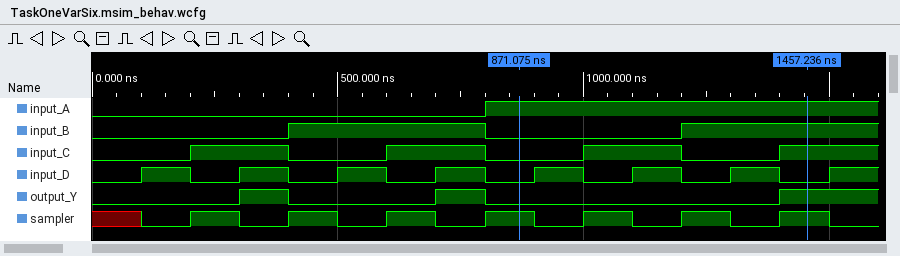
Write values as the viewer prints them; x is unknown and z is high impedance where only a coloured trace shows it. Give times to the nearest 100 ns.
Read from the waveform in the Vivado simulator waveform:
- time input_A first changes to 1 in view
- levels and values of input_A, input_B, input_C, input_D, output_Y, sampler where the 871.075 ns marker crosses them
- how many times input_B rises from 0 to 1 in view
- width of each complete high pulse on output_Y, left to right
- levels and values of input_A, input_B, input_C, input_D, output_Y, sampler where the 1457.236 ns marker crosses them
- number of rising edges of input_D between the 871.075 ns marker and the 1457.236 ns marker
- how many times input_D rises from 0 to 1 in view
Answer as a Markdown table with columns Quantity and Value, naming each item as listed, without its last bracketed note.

| Quantity | Value |
|---|---|
| time input_A first changes to 1 in view | 800 ns |
| levels and values of input_A, input_B, input_C, input_D, output_Y, sampler where the 871.075 ns marker crosses them | input_A=1, input_B=0, input_C=0, input_D=0, output_Y=0, sampler=1 |
| how many times input_B rises from 0 to 1 in view | 2 |
| width of each complete high pulse on output_Y, left to right | 100 ns, 100 ns |
| levels and values of input_A, input_B, input_C, input_D, output_Y, sampler where the 1457.236 ns marker crosses them | input_A=1, input_B=1, input_C=1, input_D=0, output_Y=1, sampler=1 |
| number of rising edges of input_D between the 871.075 ns marker and the 1457.236 ns marker | 3 |
| how many times input_D rises from 0 to 1 in view | 8 |
